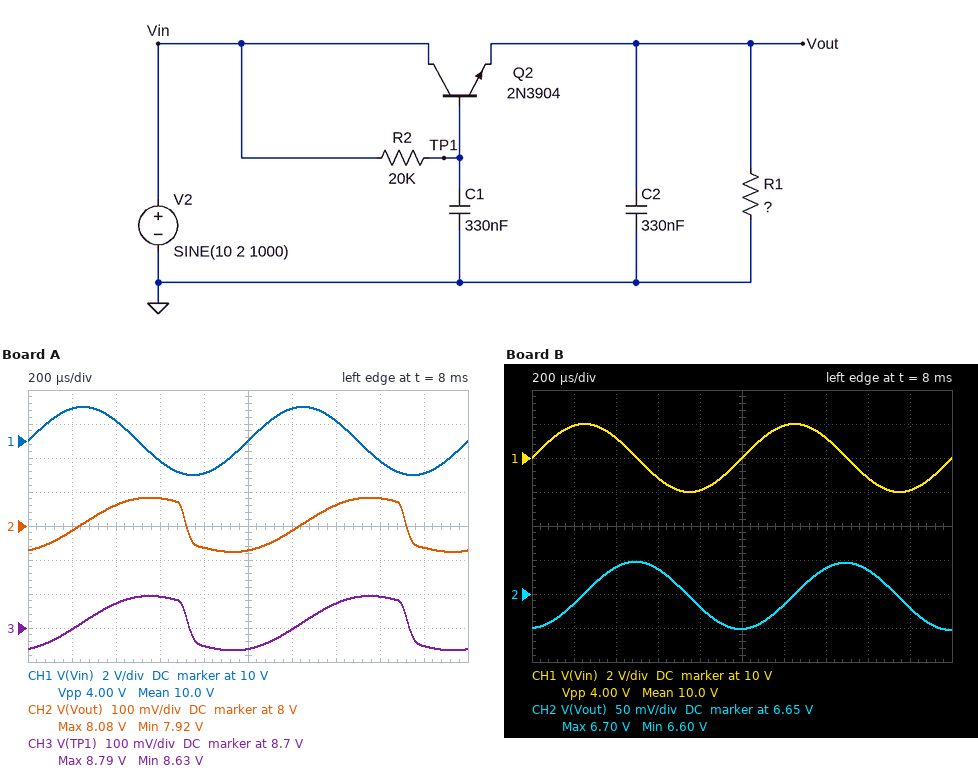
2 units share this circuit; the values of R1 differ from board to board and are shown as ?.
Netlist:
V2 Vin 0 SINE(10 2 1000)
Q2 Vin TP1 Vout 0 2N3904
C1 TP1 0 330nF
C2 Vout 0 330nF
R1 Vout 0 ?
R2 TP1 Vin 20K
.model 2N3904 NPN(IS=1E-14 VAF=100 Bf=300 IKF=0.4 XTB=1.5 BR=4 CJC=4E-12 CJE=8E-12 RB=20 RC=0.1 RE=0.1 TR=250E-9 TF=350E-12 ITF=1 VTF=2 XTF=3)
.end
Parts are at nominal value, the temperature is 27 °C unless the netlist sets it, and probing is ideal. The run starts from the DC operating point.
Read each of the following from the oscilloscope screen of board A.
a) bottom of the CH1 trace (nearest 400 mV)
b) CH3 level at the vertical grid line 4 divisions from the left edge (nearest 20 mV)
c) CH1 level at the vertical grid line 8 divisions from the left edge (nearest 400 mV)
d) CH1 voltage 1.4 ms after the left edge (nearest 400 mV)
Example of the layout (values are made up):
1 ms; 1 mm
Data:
8.0 V; 8.64 V; 8.8 V; 11.2 V
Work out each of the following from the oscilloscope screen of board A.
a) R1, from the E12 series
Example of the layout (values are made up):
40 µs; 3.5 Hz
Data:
1 kΩ
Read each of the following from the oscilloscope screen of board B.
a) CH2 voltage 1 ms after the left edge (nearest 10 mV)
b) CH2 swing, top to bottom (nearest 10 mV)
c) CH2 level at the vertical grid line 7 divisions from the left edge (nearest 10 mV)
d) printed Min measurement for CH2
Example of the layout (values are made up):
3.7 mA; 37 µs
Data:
6.60 V; 100 mV; 6.69 V; 6.60 V
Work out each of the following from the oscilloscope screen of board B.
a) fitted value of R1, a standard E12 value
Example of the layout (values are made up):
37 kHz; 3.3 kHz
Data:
180 Ω
